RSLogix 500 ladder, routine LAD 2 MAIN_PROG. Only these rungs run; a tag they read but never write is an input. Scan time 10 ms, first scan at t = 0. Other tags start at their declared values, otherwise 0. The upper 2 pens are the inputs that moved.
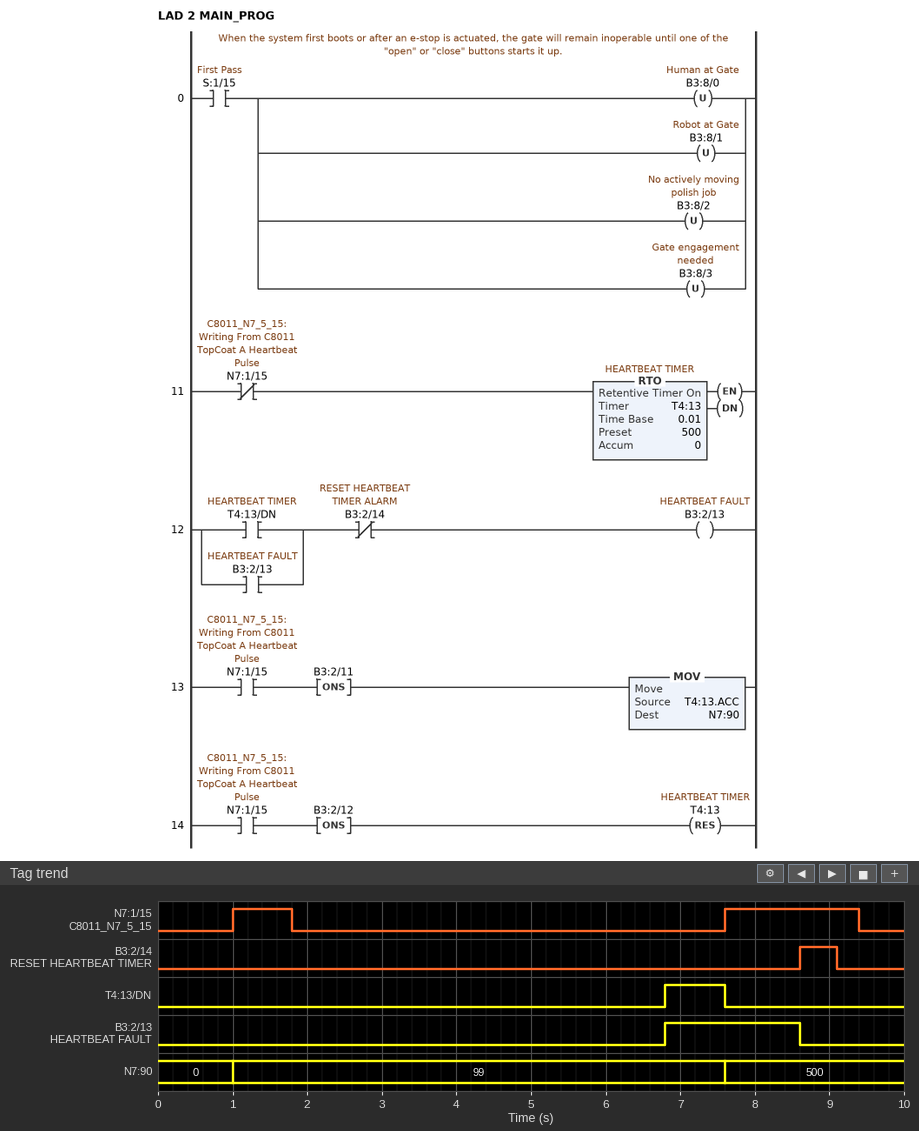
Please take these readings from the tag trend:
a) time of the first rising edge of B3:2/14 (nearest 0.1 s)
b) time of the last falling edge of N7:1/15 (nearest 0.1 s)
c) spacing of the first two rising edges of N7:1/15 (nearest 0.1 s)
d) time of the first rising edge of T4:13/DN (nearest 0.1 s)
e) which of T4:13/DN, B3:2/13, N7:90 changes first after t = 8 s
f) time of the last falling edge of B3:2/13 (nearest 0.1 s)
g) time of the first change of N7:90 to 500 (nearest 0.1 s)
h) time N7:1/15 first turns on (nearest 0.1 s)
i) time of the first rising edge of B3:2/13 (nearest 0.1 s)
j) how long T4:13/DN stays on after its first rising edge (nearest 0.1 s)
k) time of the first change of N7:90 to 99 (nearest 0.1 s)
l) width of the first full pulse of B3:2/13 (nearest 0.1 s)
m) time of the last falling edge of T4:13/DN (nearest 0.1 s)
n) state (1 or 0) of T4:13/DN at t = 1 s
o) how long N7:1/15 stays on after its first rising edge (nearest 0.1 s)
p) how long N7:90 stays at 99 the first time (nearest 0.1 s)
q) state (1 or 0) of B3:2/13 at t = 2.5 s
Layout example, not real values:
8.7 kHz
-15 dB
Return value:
8.6 s
9.4 s
6.6 s
6.8 s
B3:2/13
8.6 s
7.6 s
1.0 s
6.8 s
0.8 s
1.0 s
1.8 s
7.6 s
0
0.8 s
6.6 s
0
